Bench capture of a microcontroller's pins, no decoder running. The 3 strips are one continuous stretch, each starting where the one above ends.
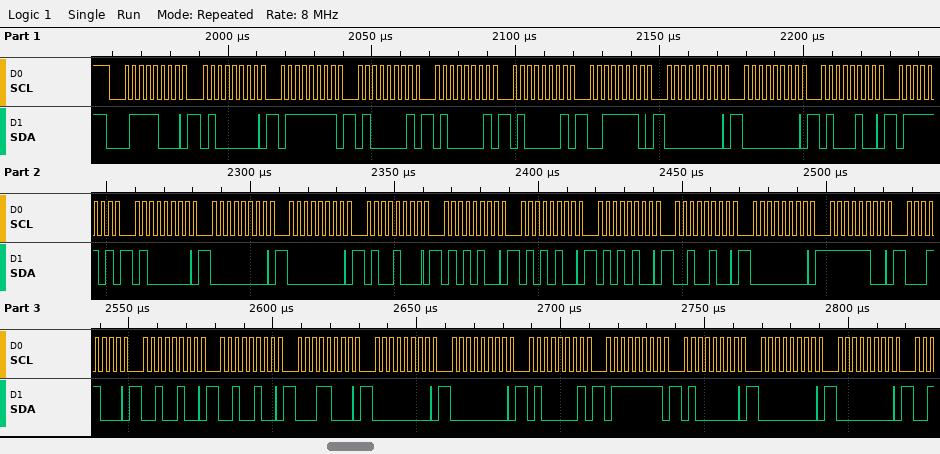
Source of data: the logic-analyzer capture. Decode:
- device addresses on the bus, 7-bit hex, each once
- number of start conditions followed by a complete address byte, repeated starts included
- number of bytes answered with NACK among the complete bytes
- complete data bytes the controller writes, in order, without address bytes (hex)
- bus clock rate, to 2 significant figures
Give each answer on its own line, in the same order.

0x3C
1
0
40 7F 41 41 41 3E 00 00 44 7D 40 00 00 48 54 54 54 24 00 FC 18 24 24 18 00 00 41 7F 40 00 00
400 kHz
